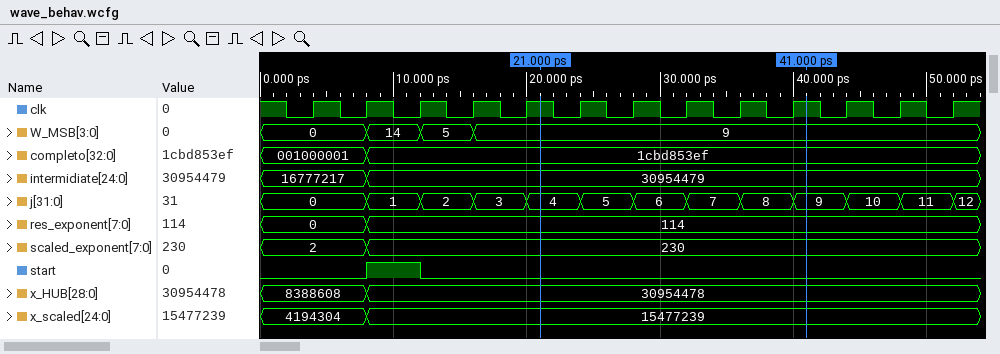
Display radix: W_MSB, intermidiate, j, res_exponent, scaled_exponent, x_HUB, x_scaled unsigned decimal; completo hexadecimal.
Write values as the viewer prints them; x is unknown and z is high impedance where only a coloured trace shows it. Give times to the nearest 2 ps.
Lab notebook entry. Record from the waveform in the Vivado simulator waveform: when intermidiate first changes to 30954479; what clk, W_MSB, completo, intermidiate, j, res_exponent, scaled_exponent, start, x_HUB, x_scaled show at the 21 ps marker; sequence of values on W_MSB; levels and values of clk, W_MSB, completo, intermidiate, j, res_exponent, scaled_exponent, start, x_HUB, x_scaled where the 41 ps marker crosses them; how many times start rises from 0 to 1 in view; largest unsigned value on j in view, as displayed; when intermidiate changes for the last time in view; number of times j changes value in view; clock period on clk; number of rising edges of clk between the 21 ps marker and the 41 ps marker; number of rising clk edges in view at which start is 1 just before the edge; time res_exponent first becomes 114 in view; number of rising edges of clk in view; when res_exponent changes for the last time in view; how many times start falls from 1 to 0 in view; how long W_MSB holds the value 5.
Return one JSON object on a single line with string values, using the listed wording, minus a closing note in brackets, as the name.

{"when intermidiate first changes to 30954479": "8 ps", "what clk, W_MSB, completo, intermidiate, j, res_exponent, scaled_exponent, start, x_HUB, x_scaled show at the 21 ps marker": "clk=1, W_MSB=9, completo=1cbd853ef, intermidiate=30954479, j=4, res_exponent=114, scaled_exponent=230, start=0, x_HUB=30954478, x_scaled=15477239", "sequence of values on W_MSB": "0, 14, 5, 9", "levels and values of clk, W_MSB, completo, intermidiate, j, res_exponent, scaled_exponent, start, x_HUB, x_scaled where the 41 ps marker crosses them": "clk=1, W_MSB=9, completo=1cbd853ef, intermidiate=30954479, j=9, res_exponent=114, scaled_exponent=230, start=0, x_HUB=30954478, x_scaled=15477239", "how many times start rises from 0 to 1 in view": "1", "largest unsigned value on j in view, as displayed": "12", "when intermidiate changes for the last time in view": "8 ps", "number of times j changes value in view": "12", "clock period on clk": "4 ps", "number of rising edges of clk between the 21 ps marker and the 41 ps marker": "5", "number of rising clk edges in view at which start is 1 just before the edge": "1", "time res_exponent first becomes 114 in view": "8 ps", "number of rising edges of clk in view": "13", "when res_exponent changes for the last time in view": "8 ps", "how many times start falls from 1 to 0 in view": "1", "how long W_MSB holds the value 5": "4 ps"}
